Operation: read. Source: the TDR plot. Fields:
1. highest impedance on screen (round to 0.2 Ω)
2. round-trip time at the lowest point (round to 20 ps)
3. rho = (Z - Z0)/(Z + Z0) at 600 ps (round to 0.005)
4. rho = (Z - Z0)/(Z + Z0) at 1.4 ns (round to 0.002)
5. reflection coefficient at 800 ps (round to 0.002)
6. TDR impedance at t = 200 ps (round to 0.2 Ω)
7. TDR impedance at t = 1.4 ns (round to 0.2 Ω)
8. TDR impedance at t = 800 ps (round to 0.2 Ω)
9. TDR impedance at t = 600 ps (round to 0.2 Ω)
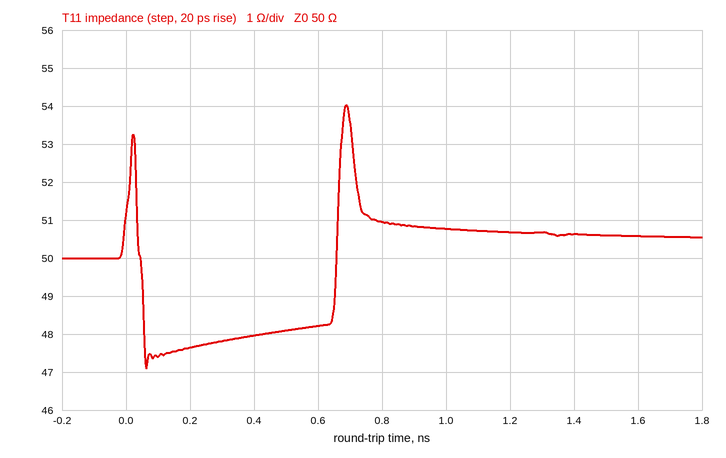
54.0 Ω
60 ps
-0.020
+0.006
+0.010
47.6 Ω
50.6 Ω
51.0 Ω
48.2 Ω
